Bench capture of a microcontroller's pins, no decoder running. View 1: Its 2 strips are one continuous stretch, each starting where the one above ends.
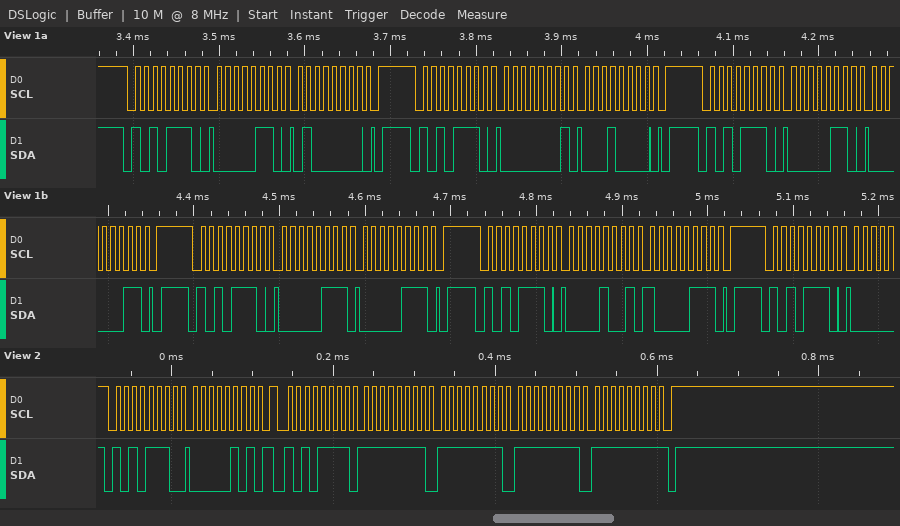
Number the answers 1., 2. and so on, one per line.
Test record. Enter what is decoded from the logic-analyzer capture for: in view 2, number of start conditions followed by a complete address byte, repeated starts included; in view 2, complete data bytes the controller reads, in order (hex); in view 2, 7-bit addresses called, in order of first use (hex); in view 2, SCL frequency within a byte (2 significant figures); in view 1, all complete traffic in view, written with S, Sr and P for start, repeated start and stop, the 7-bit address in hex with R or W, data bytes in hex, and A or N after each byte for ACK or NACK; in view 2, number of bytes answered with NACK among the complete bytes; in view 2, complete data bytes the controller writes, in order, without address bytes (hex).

1. 2
2. FF FF FF FF
3. 0x57
4. 100 kHz
5. S 57W A 06 A 40 A P S 57W A 01 A 10 A P S 57W A 06 A 03 A P S 57W A 07 A 07 A P S 57W A 09 A 87 A P S 57W A
6. 1
7. 05
